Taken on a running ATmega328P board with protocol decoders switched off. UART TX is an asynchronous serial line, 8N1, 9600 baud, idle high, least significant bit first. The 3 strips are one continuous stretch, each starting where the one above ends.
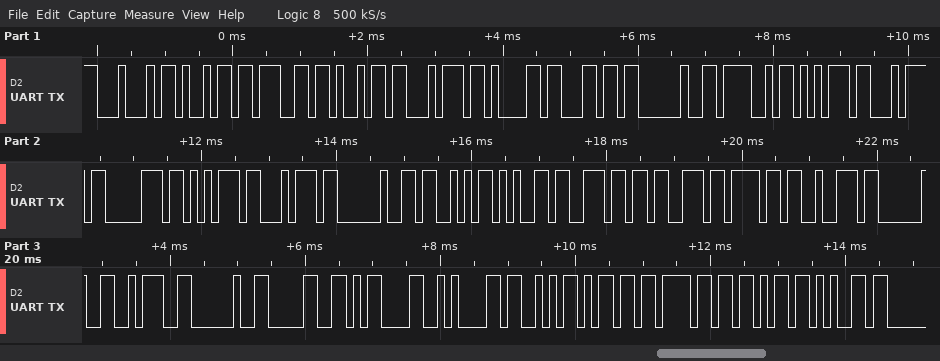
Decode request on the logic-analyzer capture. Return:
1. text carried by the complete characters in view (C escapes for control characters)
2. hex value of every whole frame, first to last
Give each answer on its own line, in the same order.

"Digital Output Sensor : 0\r\nSmoke"
44 69 67 69 74 61 6C 20 4F 75 74 70 75 74 20 53 65 6E 73 6F 72 20 3A 20 30 0D 0A 53 6D 6F 6B 65
